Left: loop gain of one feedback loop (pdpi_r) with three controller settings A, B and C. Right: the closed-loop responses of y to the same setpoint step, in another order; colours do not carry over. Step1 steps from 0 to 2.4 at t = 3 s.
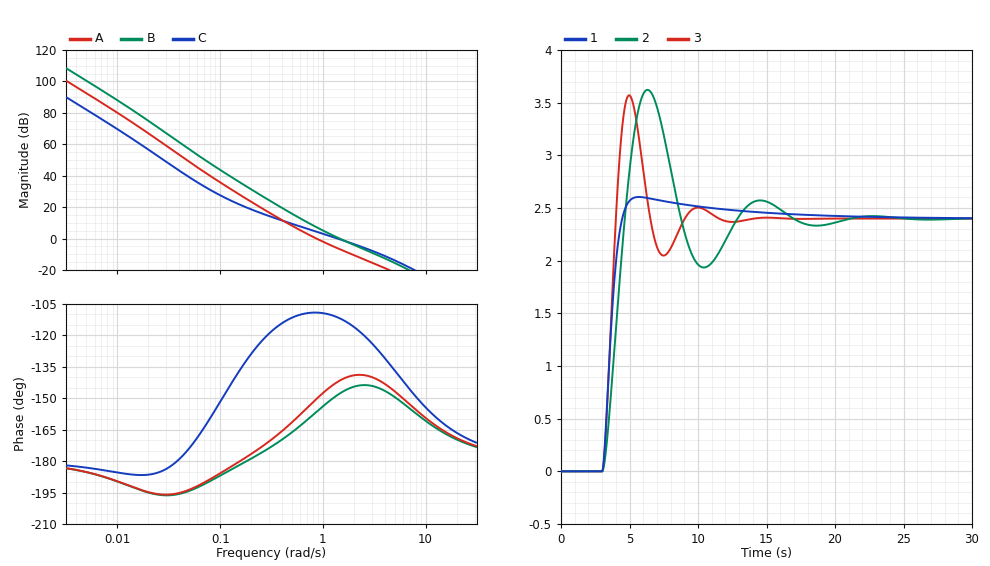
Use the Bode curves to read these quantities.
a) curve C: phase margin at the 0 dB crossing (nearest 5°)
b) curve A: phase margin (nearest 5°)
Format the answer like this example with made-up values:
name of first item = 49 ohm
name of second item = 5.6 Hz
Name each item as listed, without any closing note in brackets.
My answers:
curve C: phase margin at the 0 dB crossing = 70°
curve A: phase margin = 30°
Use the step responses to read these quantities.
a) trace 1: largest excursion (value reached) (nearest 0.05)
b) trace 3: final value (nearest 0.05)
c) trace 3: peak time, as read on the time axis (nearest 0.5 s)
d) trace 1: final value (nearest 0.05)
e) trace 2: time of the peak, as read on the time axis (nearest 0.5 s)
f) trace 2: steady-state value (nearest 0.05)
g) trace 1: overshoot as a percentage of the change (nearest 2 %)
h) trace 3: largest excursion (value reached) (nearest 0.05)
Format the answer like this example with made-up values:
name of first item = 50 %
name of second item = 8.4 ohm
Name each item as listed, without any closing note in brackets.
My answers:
trace 1: largest excursion (value reached) = 2.60
trace 3: final value = 2.40
trace 3: peak time, as read on the time axis = 5.0 s
trace 1: final value = 2.40
trace 2: time of the peak, as read on the time axis = 6.5 s
trace 2: steady-state value = 2.40
trace 1: overshoot as a percentage of the change = 8 %
trace 3: largest excursion (value reached) = 3.55
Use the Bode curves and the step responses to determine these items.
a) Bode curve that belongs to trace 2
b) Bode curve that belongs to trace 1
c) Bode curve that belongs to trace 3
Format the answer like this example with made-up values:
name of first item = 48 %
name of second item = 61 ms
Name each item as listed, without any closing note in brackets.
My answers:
Bode curve that belongs to trace 2 = A
Bode curve that belongs to trace 1 = C
Bode curve that belongs to trace 3 = B
